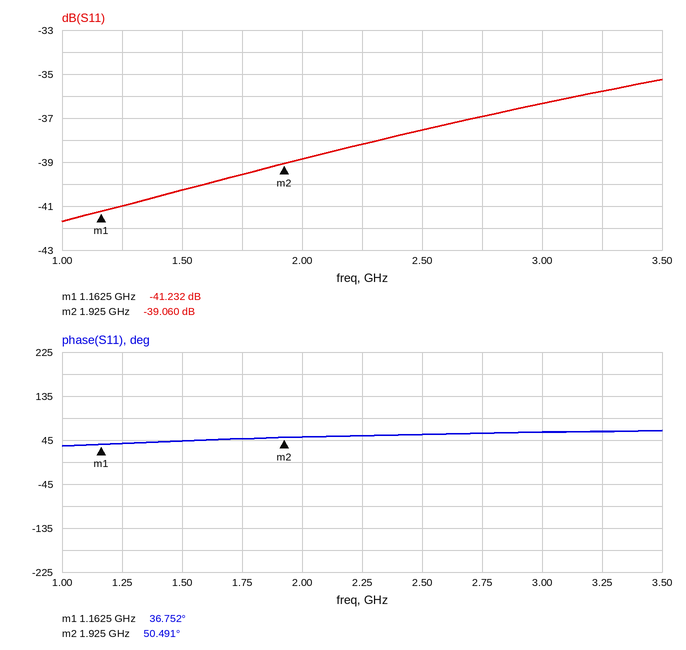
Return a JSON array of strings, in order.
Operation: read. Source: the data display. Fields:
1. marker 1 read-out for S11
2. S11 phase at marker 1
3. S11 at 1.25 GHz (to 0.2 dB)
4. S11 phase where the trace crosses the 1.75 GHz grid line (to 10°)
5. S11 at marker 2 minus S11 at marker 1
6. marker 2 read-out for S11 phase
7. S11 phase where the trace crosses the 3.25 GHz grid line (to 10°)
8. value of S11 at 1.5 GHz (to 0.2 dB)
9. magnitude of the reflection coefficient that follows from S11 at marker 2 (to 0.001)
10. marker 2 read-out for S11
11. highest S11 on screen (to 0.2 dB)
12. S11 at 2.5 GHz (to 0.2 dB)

["-41.232 dB", "36.752°", "-41.0 dB", "50°", "2.172 dB", "50.491°", "60°", "-40.2 dB", "0.011", "-39.060 dB", "-35.2 dB", "-37.6 dB"]
